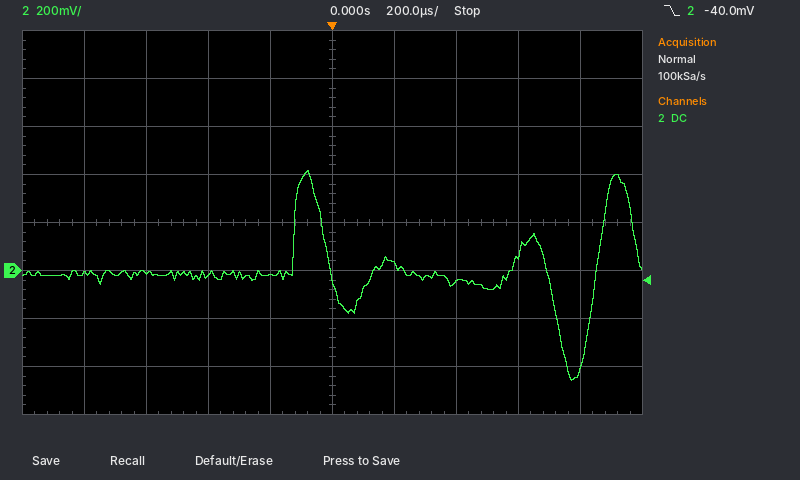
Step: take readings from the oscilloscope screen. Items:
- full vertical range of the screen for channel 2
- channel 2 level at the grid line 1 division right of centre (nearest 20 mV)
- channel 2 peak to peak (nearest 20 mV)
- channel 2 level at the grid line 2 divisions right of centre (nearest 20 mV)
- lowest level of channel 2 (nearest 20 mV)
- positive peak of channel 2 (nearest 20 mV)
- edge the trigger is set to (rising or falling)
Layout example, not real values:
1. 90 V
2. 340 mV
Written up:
1. 1.6 V
2. 20 mV
3. 880 mV
4. -40 mV
5. -460 mV
6. 420 mV
7. falling
